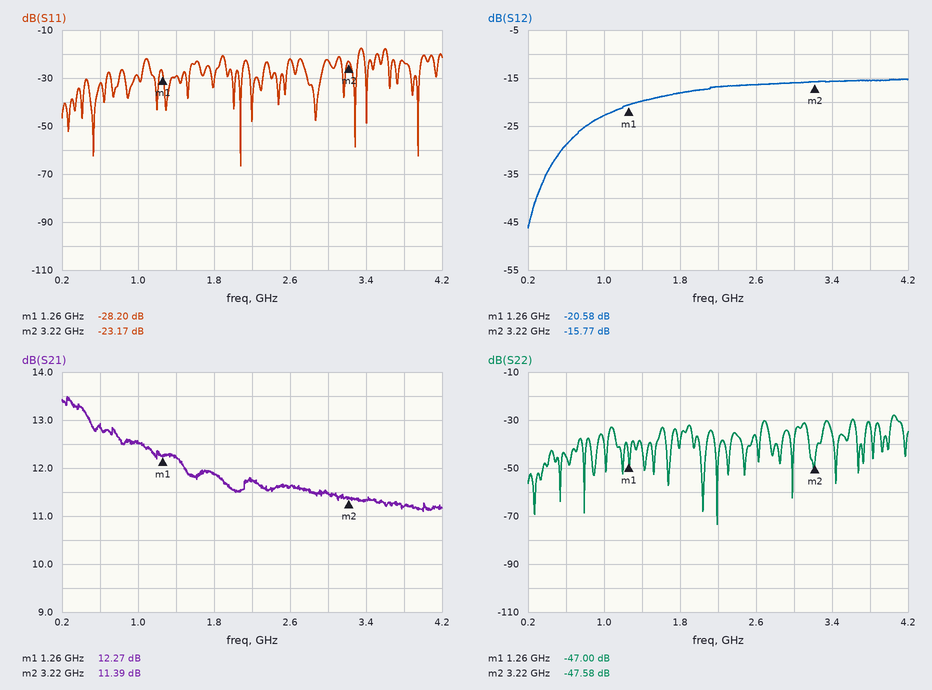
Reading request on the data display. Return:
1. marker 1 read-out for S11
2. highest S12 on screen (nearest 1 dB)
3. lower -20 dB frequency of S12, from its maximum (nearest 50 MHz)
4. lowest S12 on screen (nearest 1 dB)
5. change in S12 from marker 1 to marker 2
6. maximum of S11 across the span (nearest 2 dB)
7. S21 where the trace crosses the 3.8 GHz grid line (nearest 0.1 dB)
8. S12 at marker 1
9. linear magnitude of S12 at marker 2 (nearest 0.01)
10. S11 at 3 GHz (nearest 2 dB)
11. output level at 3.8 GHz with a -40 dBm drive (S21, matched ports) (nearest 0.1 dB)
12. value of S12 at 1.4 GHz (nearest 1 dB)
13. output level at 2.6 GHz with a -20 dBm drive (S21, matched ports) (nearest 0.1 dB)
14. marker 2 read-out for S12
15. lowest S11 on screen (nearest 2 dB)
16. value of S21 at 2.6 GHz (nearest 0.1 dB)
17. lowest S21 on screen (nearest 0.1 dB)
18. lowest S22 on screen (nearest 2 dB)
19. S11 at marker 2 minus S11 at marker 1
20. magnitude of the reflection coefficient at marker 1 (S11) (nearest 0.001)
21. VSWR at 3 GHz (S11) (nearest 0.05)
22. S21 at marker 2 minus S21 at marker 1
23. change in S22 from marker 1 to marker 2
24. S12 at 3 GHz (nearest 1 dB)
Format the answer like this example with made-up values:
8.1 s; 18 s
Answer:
-28.20 dB; -15 dB; 400 MHz; -46 dB; 4.81 dB; -18 dB; 11.2 dB; -20.58 dB; 0.16; -22 dB; -28.8 dBm; -20 dB; -8.4 dBm; -15.77 dB; -66 dB; 11.6 dB; 11.1 dB; -74 dB; 5.03 dB; 0.039; 1.15; -0.88 dB; -0.58 dB; -16 dB
